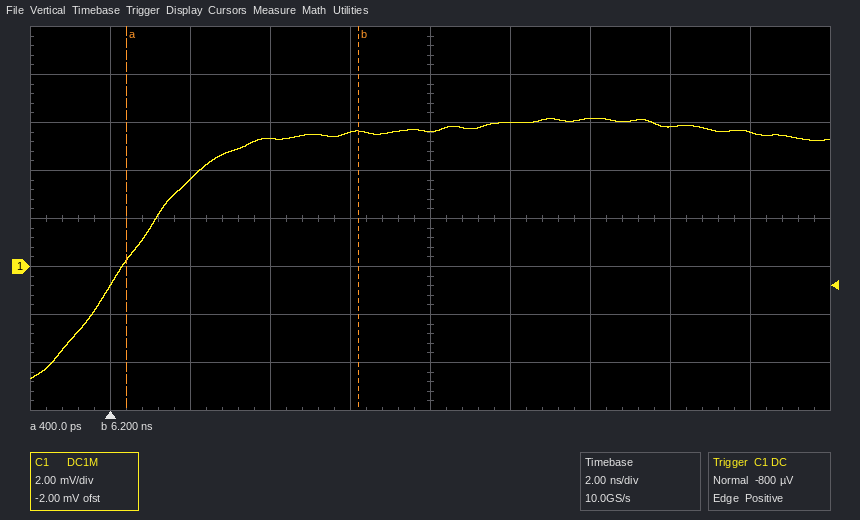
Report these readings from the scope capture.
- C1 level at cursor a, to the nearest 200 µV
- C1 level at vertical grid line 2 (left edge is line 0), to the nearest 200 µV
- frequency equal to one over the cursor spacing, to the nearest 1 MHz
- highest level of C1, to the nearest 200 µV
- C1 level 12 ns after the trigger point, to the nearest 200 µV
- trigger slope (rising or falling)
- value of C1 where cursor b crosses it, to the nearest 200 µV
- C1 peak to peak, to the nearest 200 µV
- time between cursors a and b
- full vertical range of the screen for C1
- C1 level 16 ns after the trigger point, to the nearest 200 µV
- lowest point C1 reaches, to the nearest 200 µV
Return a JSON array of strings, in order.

["200 µV", "3.6 mV", "172 MHz", "6.2 mV", "6.2 mV", "rising", "5.6 mV", "10.8 mV", "5.8 ns", "16 mV", "5.6 mV", "-4.6 mV"]
